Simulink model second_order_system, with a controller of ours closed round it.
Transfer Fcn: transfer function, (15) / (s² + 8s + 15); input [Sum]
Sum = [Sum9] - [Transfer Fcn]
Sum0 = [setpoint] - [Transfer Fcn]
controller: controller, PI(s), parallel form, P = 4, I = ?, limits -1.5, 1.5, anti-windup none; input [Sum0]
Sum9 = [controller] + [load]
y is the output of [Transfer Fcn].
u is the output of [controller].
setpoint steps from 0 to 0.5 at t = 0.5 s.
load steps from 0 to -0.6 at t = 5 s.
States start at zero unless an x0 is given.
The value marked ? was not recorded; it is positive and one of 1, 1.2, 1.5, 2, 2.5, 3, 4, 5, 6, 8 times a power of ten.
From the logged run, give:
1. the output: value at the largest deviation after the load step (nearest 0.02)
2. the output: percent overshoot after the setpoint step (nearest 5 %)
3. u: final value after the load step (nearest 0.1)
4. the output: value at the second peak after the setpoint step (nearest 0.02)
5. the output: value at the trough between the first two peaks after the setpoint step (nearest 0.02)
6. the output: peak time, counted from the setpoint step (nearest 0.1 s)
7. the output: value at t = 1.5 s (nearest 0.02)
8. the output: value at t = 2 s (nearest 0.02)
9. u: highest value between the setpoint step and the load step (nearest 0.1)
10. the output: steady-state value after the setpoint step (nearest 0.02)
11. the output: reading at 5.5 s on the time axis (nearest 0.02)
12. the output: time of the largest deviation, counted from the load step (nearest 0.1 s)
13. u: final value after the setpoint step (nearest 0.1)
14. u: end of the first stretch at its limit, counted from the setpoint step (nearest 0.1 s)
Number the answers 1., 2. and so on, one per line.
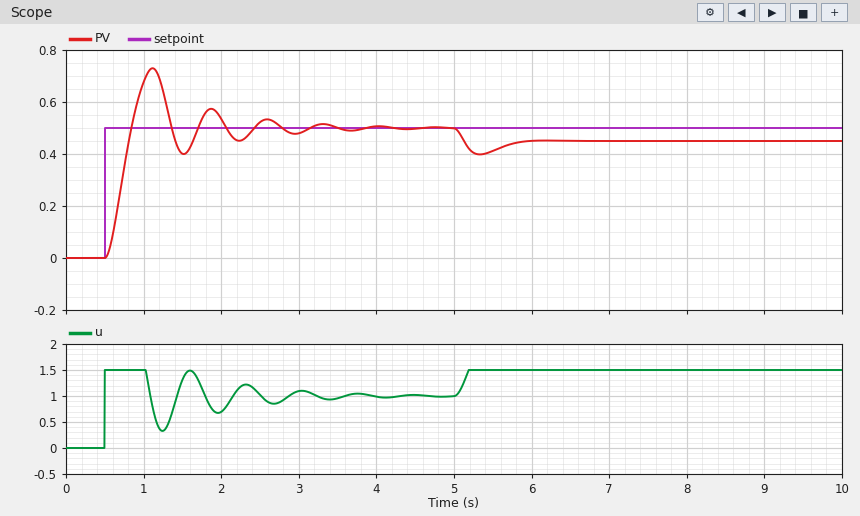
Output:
1. 0.40
2. 45 %
3. 1.5
4. 0.58
5. 0.40
6. 0.6 s
7. 0.40
8. 0.54
9. 1.5
10. 0.50
11. 0.42
12. 0.3 s
13. 1.0
14. 0.5 s
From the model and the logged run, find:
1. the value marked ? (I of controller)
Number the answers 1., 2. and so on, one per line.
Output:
1. 30
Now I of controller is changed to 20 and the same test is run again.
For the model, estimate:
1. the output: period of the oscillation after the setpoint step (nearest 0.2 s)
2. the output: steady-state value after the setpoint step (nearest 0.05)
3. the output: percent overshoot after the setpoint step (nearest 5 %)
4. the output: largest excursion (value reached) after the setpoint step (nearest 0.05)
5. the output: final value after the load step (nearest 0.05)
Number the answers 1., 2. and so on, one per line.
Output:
1. 0.8 s
2. 0.50
3. 35 %
4. 0.70
5. 0.45
